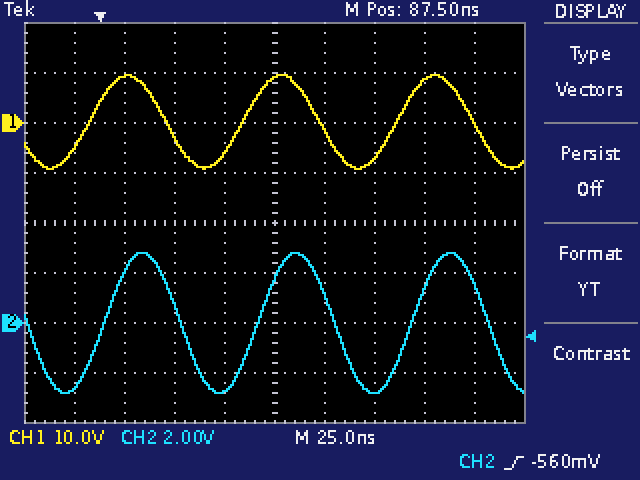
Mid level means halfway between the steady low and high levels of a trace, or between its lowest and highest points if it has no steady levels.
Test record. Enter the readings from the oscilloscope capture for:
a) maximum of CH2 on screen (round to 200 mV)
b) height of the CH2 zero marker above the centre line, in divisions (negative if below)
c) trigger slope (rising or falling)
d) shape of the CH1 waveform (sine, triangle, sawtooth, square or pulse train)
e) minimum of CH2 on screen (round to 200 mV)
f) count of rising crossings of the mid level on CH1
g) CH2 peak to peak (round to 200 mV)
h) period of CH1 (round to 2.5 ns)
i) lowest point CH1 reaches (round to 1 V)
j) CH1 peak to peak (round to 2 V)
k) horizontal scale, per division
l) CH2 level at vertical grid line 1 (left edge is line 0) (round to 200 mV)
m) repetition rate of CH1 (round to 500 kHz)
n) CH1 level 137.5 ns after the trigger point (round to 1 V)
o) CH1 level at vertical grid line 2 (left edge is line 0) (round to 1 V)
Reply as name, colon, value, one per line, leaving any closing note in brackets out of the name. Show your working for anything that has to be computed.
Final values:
maximum of CH2 on screen: 2.8 V
height of the CH2 zero marker above the centre line, in divisions: -2.0 div
trigger slope: rising
shape of the CH1 waveform: sine
minimum of CH2 on screen: -2.8 V
count of rising crossings of the mid level on CH1: 3
CH2 peak to peak: 2.8 V − (-2.8 V) = 5.6 V
period of CH1: 77.5 ns
lowest point CH1 reaches: -9 V
CH1 peak to peak: 18 V
horizontal scale, per division: 25 ns
CH2 level at vertical grid line 1 (left edge is line 0): -2.6 V
repetition rate of CH1: 1 / 77.5 ns ≈ 12.9 MHz, so 13.0 MHz to the nearest 500 kHz
CH1 level 137.5 ns after the trigger point: -7 V
CH1 level at vertical grid line 2 (left edge is line 0): 9 V
